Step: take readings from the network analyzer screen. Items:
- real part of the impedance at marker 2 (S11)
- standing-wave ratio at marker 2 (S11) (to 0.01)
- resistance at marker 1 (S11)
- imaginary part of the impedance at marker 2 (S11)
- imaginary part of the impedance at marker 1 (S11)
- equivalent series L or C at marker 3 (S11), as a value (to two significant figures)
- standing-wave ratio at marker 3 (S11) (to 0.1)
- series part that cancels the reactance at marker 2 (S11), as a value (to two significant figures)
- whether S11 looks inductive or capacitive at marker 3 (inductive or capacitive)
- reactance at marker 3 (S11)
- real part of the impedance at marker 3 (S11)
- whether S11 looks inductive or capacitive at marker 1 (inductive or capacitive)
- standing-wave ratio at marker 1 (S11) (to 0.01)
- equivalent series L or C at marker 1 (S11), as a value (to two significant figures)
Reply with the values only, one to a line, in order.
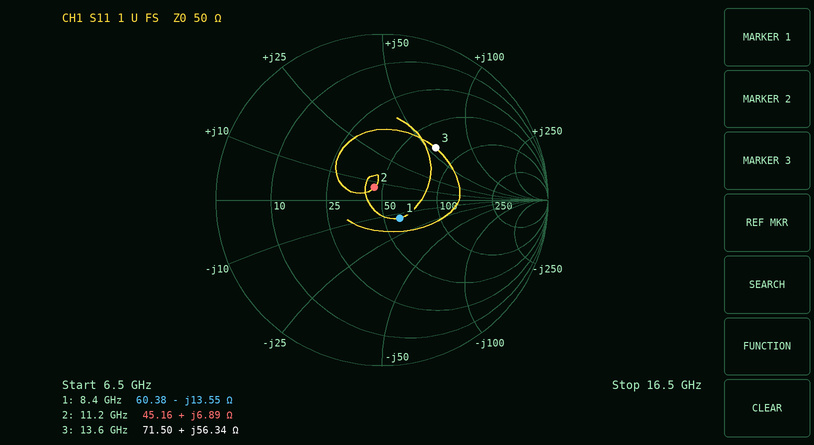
45.16 Ω
1.19
60.38 Ω
+6.89 Ω
-13.55 Ω
660 pH
2.6
2.1 pF
inductive
+56.34 Ω
71.50 Ω
capacitive
1.36
1.4 pF
